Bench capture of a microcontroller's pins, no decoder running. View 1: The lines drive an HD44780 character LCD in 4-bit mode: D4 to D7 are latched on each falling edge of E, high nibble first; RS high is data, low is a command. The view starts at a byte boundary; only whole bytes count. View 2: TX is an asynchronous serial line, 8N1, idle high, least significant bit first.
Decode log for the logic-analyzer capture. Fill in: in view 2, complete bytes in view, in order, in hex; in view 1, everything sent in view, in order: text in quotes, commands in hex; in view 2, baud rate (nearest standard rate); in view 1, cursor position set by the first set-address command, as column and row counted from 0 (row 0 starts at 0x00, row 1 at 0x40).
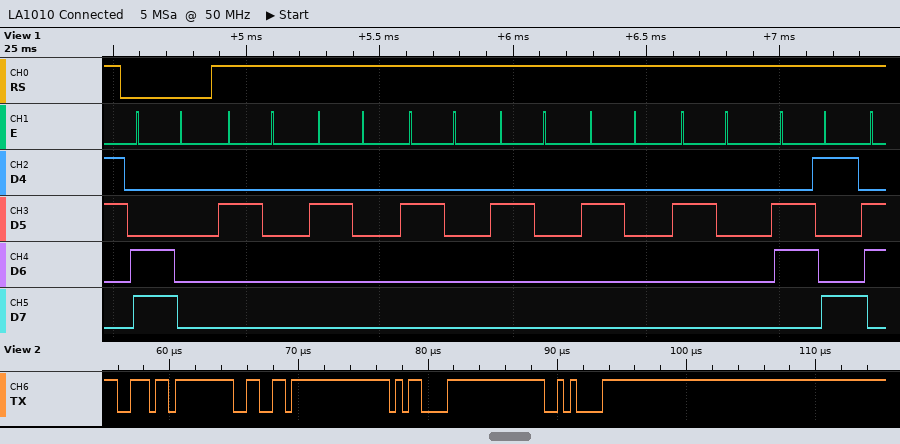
6E 66 0D 0A
0xC0 "      i"
2000000 baud
column 0, row 1
